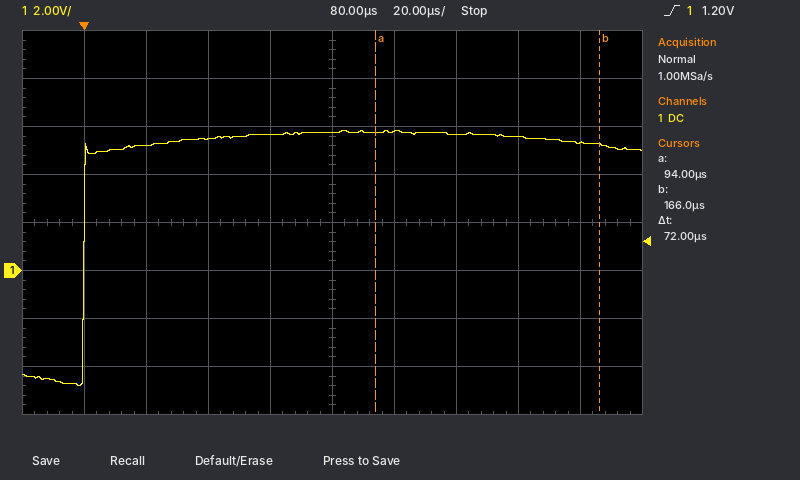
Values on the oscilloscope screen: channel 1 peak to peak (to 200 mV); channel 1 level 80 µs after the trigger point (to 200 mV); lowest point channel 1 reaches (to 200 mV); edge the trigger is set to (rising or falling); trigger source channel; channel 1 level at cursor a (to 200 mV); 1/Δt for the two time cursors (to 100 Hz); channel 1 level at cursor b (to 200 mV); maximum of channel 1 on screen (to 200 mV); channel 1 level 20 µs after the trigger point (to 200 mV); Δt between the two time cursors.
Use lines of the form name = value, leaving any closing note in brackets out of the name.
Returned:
channel 1 peak to peak = 10.6 V
channel 1 level 80 µs after the trigger point = 5.8 V
lowest point channel 1 reaches = -4.8 V
edge the trigger is set to = rising
trigger source channel = channel 1
channel 1 level at cursor a = 5.8 V
1/Δt for the two time cursors = 13.9 kHz
channel 1 level at cursor b = 5.2 V
maximum of channel 1 on screen = 5.8 V
channel 1 level 20 µs after the trigger point = 5.2 V
Δt between the two time cursors = 72 µs
